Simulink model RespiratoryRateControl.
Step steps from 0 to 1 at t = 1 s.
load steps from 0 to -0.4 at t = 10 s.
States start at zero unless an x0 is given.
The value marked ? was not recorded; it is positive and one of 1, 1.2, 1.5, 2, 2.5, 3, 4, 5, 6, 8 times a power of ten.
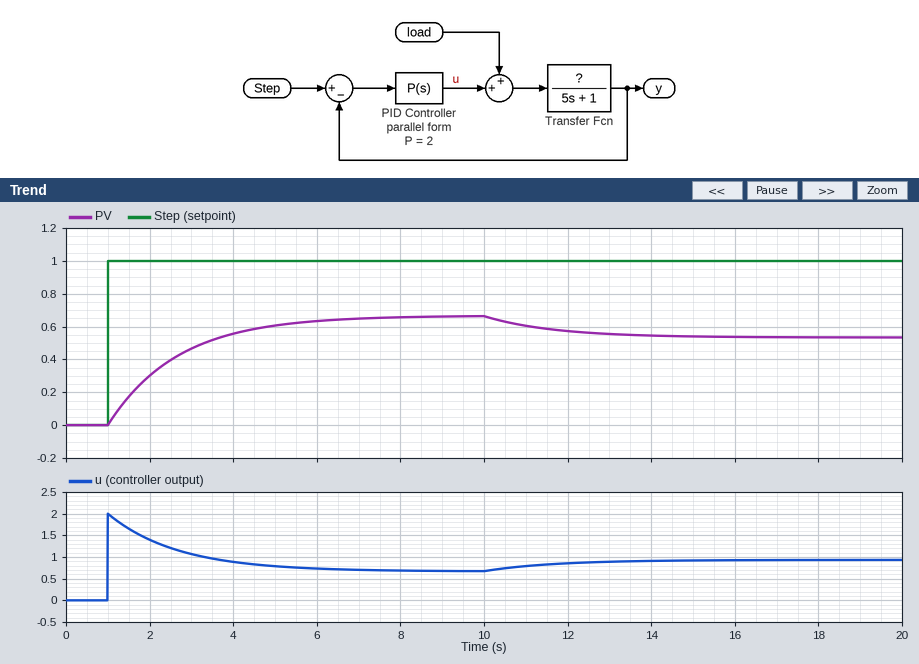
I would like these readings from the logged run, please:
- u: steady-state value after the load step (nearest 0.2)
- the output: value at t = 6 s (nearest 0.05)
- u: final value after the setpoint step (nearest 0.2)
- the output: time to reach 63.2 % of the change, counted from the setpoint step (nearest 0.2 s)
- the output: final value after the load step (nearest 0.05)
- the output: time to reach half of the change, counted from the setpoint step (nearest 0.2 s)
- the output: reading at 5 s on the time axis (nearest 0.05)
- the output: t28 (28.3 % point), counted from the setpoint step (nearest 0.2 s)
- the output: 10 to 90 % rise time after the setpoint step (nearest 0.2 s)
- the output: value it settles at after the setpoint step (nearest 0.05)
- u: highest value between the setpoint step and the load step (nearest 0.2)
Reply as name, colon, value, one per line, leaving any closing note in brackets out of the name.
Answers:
u: steady-state value after the load step: 1.0
the output: value at t = 6 s: 0.65
u: final value after the setpoint step: 0.6
the output: time to reach 63.2 % of the change, counted from the setpoint step: 1.6 s
the output: final value after the load step: 0.55
the output: time to reach half of the change, counted from the setpoint step: 1.2 s
the output: reading at 5 s on the time axis: 0.60
the output: t28 (28.3 % point), counted from the setpoint step: 0.6 s
the output: 10 to 90 % rise time after the setpoint step: 3.6 s
the output: value it settles at after the setpoint step: 0.65
u: highest value between the setpoint step and the load step: 2.0
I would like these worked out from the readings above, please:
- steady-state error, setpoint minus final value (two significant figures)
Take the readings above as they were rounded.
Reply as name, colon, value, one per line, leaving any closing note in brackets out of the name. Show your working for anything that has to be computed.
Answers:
steady-state error, setpoint minus final value: 1 - 0.65 = 0.35
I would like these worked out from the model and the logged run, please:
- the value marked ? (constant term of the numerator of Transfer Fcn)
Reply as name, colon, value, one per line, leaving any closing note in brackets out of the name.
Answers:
the value marked ?: 1
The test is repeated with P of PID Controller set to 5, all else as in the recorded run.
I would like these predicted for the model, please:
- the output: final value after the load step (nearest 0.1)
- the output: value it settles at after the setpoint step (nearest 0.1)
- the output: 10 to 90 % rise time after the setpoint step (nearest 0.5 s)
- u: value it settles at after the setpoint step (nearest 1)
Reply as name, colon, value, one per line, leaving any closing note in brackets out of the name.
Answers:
the output: final value after the load step: 0.8
the output: value it settles at after the setpoint step: 0.8
the output: 10 to 90 % rise time after the setpoint step: 2.0 s
u: value it settles at after the setpoint step: 1
